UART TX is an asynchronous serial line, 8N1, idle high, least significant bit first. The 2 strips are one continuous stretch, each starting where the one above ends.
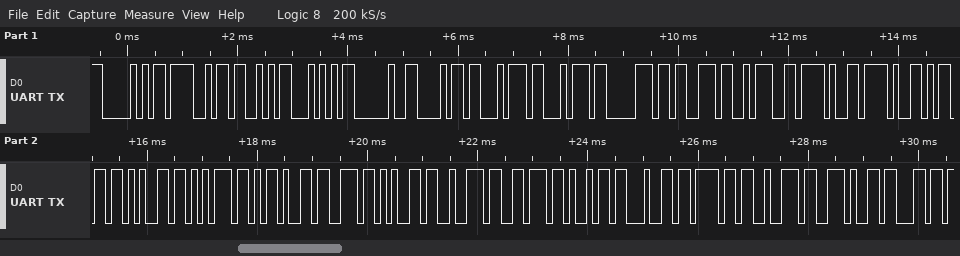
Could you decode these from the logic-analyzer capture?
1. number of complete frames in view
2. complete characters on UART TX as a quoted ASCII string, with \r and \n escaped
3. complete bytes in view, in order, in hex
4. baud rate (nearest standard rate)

27
"POST https://meu-servidor.c"
50 4F 53 54 20 68 74 74 70 73 3A 2F 2F 6D 65 75 2D 73 65 72 76 69 64 6F 72 2E 63
9600 baud
